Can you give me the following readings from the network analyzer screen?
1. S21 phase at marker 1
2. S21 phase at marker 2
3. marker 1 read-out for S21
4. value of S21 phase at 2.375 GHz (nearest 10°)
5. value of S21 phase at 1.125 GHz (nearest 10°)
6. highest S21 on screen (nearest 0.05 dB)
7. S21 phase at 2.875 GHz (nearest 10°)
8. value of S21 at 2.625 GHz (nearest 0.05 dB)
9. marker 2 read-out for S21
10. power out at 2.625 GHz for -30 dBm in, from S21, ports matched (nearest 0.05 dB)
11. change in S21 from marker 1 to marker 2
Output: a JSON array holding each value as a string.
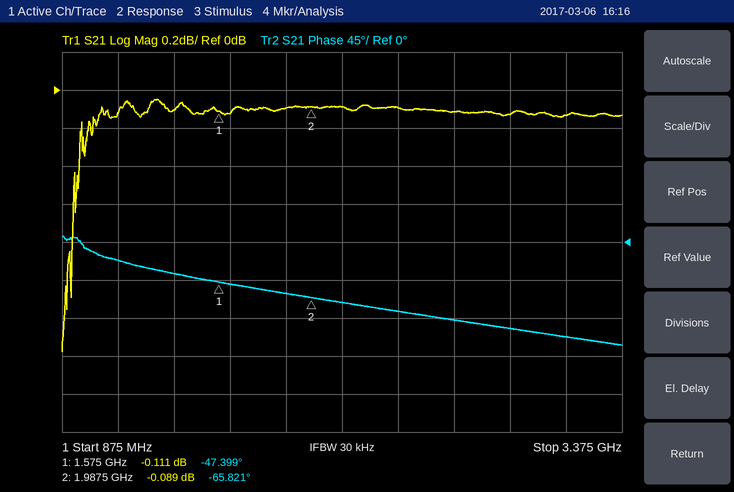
["-47.399°", "-65.821°", "-0.111 dB", "-80°", "-20°", "-0.05 dB", "-100°", "-0.10 dB", "-0.089 dB", "-30.10 dBm", "0.022 dB"]
